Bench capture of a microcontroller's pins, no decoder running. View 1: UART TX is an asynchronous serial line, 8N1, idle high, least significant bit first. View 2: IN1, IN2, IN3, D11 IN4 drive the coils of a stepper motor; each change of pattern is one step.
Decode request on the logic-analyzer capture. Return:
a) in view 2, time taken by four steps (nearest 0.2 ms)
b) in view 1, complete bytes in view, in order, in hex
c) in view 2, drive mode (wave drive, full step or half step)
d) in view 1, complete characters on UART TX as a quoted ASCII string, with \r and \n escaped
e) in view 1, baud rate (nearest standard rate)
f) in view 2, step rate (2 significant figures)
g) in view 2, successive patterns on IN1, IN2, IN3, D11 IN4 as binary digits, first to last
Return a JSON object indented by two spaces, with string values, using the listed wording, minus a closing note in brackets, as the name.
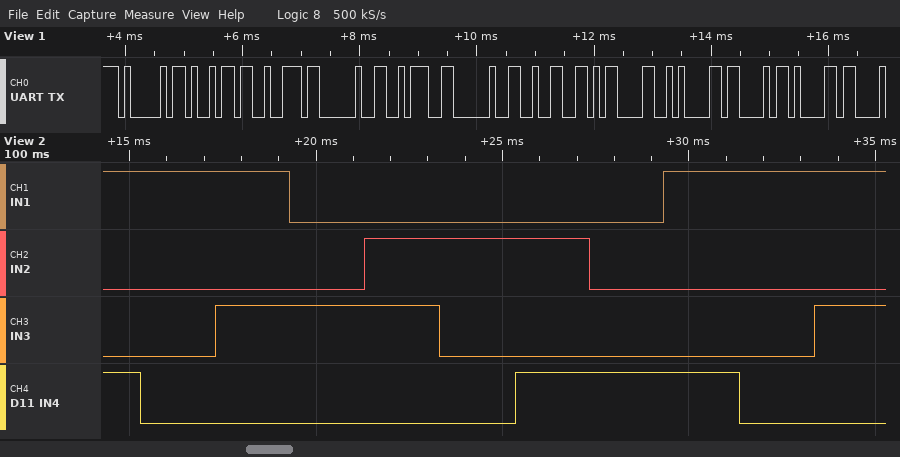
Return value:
{
  "in view 2, time taken by four steps": "8.0 ms",
  "in view 1, complete bytes in view, in order, in hex": "41 69 72 20 3A 20 32 0D 0A 43 61",
  "in view 2, drive mode": "half step",
  "in view 1, complete characters on UART TX as a quoted ASCII string, with \\r and \\n escaped": "\"Air : 2\\r\\nCa\"",
  "in view 1, baud rate": "9600 baud",
  "in view 2, step rate": "500 steps/s",
  "in view 2, successive patterns on IN1, IN2, IN3, D11 IN4 as binary digits, first to last": "1001 1000 1010 0010 0110 0100 0101 0001 1001 1000 1010"
}
